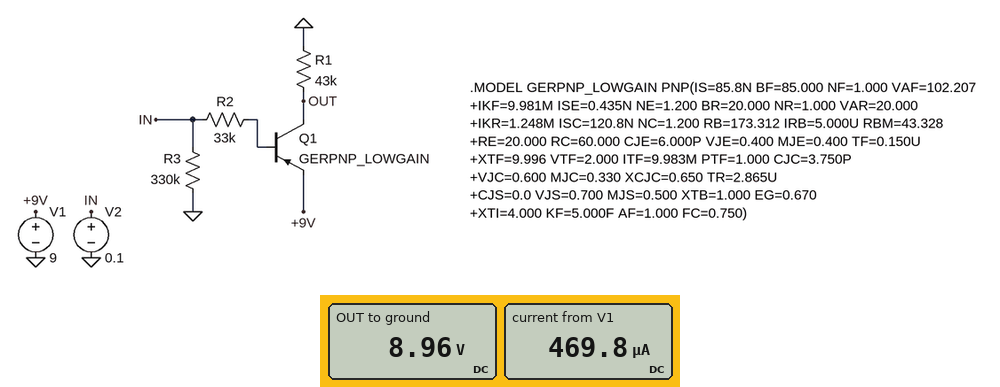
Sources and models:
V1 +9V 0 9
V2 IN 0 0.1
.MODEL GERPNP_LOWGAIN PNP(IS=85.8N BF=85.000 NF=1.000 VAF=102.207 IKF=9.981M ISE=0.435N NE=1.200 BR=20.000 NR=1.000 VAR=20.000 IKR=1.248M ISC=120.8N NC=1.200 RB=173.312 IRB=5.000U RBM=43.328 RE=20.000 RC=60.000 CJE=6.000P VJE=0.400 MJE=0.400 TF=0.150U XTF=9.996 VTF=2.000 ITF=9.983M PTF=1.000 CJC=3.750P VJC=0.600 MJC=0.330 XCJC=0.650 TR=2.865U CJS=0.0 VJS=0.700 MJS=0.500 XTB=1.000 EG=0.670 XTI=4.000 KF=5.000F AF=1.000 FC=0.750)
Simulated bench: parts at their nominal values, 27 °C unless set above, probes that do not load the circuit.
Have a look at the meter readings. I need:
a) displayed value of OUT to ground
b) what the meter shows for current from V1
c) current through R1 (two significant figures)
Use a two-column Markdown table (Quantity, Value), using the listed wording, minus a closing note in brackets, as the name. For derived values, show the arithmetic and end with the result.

| Quantity | Value |
|---|---|
| displayed value of OUT to ground | 8.96 V |
| what the meter shows for current from V1 | 469.8 µA |
| current through R1 | (8.96 V) / 43 kΩ = 210 µA |
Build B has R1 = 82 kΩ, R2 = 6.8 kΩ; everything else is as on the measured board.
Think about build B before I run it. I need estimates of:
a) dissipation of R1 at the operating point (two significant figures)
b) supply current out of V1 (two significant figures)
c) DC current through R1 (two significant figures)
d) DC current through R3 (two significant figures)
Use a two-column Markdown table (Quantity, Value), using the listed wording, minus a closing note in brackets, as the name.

| Quantity | Value |
|---|---|
| dissipation of R1 at the operating point | 980 µW |
| supply current out of V1 | 1.4 mA |
| DC current through R1 | 110 µA |
| DC current through R3 | 300 nA |
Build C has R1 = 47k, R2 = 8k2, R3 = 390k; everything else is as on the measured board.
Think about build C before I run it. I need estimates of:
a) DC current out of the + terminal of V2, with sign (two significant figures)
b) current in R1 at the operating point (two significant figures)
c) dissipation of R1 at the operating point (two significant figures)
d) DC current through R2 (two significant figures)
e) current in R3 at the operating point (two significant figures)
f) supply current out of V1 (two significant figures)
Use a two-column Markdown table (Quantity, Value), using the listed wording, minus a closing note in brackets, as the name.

| Quantity | Value |
|---|---|
| DC current out of the + terminal of V2, with sign | -1.0 mA |
| current in R1 at the operating point | 190 µA |
| dissipation of R1 at the operating point | 1.7 mW |
| DC current through R2 | 1.0 mA |
| current in R3 at the operating point | 260 nA |
| supply current out of V1 | 1.2 mA |
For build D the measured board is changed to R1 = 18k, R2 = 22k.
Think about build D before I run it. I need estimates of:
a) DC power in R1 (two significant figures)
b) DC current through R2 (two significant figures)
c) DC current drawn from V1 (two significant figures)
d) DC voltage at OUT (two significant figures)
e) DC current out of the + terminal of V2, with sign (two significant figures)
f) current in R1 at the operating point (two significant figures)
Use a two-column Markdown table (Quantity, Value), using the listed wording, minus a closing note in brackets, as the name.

| Quantity | Value |
|---|---|
| DC power in R1 | 4.4 mW |
| DC current through R2 | 390 µA |
| DC current drawn from V1 | 890 µA |
| DC voltage at OUT | 8.9 V |
| DC current out of the + terminal of V2, with sign | -390 µA |
| current in R1 at the operating point | 500 µA |
